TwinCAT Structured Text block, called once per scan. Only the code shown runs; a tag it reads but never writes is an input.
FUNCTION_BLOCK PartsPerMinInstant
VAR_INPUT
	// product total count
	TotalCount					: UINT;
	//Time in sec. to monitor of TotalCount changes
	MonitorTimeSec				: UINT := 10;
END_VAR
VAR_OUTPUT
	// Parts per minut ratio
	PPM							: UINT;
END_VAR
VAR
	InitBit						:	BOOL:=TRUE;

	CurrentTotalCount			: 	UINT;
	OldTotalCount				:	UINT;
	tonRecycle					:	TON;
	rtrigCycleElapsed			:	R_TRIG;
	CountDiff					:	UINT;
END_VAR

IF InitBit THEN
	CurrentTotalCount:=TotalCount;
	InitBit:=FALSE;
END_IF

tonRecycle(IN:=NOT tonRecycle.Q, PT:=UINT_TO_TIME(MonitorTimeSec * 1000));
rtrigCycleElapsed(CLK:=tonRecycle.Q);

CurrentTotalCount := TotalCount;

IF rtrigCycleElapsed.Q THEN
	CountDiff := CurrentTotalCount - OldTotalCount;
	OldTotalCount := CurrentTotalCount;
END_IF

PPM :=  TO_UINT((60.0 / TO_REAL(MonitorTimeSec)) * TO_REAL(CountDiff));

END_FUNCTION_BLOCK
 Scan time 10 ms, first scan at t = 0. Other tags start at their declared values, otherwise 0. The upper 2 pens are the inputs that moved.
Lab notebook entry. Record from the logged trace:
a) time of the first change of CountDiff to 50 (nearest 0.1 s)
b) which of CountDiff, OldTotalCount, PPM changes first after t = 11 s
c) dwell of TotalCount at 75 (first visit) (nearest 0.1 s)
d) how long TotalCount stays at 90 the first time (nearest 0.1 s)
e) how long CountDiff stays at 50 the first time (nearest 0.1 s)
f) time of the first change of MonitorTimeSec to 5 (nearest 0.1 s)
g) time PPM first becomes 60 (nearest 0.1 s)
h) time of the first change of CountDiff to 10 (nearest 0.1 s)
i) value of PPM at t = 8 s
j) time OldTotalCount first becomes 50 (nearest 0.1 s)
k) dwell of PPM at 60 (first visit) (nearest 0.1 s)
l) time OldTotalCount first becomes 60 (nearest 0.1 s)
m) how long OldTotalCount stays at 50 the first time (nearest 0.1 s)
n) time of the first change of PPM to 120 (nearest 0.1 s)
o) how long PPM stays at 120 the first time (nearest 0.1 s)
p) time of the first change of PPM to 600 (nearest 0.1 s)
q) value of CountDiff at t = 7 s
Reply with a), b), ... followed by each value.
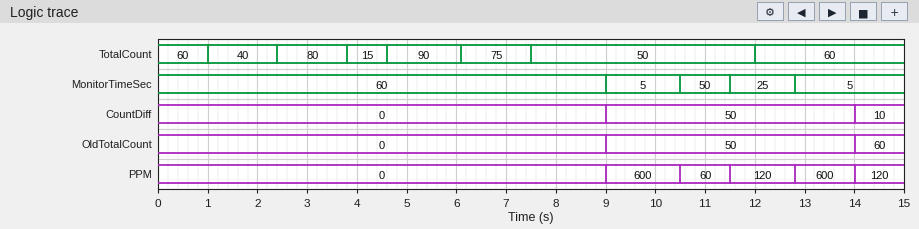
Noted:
a) 9.0 s
b) PPM
c) 1.4 s
d) 1.5 s
e) 5.0 s
f) 9.0 s
g) 10.5 s
h) 14.0 s
i) 0
j) 9.0 s
k) 1.0 s
l) 14.0 s
m) 5.0 s
n) 11.5 s
o) 1.3 s
p) 9.0 s
q) 0
